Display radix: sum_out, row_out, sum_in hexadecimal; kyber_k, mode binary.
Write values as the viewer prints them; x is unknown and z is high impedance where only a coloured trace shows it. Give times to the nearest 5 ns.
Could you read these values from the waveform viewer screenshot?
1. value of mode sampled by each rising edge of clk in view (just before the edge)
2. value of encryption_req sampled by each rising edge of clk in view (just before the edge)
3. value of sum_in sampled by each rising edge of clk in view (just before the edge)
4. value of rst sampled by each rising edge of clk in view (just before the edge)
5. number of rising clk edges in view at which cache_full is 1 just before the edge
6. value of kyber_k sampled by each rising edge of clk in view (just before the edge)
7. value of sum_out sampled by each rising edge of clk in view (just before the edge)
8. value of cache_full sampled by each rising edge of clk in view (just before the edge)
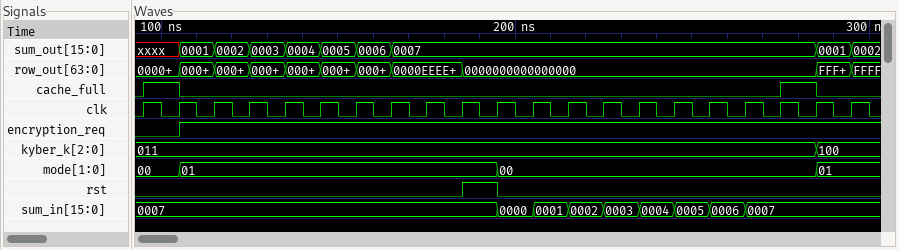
00, 00, 01, 01, 01, 01, 01, 01, 01, 01, 01, 00, 00, 00, 00, 00, 00, 00, 00, 00, 01
0 0 1 1 1 1 1 1 1 1 1 1 1 1 1 1 1 1 1 1 1
0007, 0007, 0007, 0007, 0007, 0007, 0007, 0007, 0007, 0007, 0007, 0000, 0001, 0002, 0003, 0004, 0005, 0006, 0007, 0007, 0007
0 0 0 0 0 0 0 0 0 0 1 0 0 0 0 0 0 0 0 0 0
2
011, 011, 011, 011, 011, 011, 011, 011, 011, 011, 011, 011, 011, 011, 011, 011, 011, 011, 011, 011, 100
xxxx, xxxx, 0001, 0002, 0003, 0004, 0005, 0006, 0007, 0007, 0007, 0007, 0007, 0007, 0007, 0007, 0007, 0007, 0007, 0007, 0001
0 1 0 0 0 0 0 0 0 0 0 0 0 0 0 0 0 0 0 1 0
